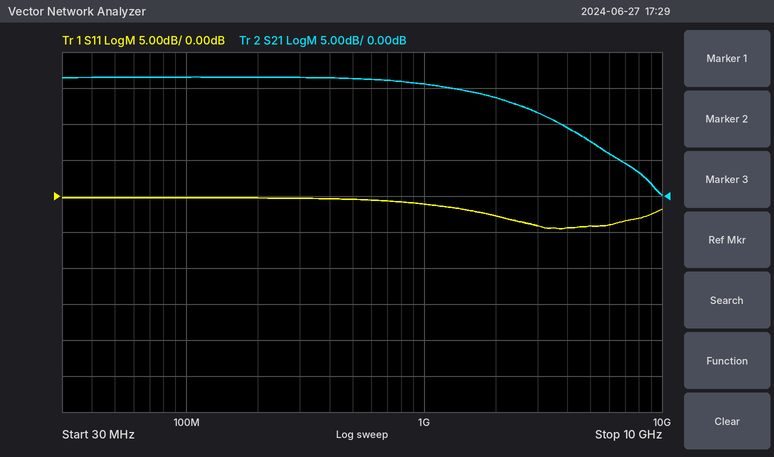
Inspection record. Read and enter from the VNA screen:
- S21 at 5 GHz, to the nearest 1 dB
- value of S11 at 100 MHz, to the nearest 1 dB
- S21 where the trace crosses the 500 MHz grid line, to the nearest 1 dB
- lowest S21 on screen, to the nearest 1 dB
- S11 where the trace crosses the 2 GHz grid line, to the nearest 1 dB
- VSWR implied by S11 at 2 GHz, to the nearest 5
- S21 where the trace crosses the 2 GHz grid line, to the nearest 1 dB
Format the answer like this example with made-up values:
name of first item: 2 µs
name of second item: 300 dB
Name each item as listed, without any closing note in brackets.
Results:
S21 at 5 GHz, to the nearest 1 dB: 8 dB
value of S11 at 100 MHz, to the nearest 1 dB: 0 dB
S21 where the trace crosses the 500 MHz grid line, to the nearest 1 dB: 16 dB
lowest S21 on screen, to the nearest 1 dB: 0 dB
S11 where the trace crosses the 2 GHz grid line, to the nearest 1 dB: -3 dB
VSWR implied by S11 at 2 GHz, to the nearest 5: 5
S21 where the trace crosses the 2 GHz grid line, to the nearest 1 dB: 14 dB
